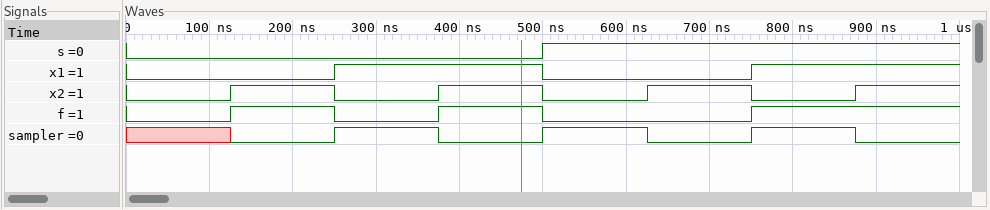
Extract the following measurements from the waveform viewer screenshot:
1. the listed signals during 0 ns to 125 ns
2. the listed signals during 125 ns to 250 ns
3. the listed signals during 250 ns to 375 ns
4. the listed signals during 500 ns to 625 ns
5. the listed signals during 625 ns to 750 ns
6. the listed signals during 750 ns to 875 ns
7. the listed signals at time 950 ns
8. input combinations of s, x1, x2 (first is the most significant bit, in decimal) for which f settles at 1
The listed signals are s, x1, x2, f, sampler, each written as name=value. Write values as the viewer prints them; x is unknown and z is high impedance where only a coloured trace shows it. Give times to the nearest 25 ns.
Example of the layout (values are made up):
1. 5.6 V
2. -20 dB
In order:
1. s=0, x1=0, x2=0, f=0, sampler=x
2. s=0, x1=0, x2=1, f=1, sampler=0
3. s=0, x1=1, x2=0, f=0, sampler=1
4. s=1, x1=0, x2=0, f=0, sampler=1
5. s=1, x1=0, x2=1, f=0, sampler=0
6. s=1, x1=1, x2=0, f=1, sampler=1
7. s=1, x1=1, x2=1, f=1, sampler=0
8. 1, 3, 6, 7
